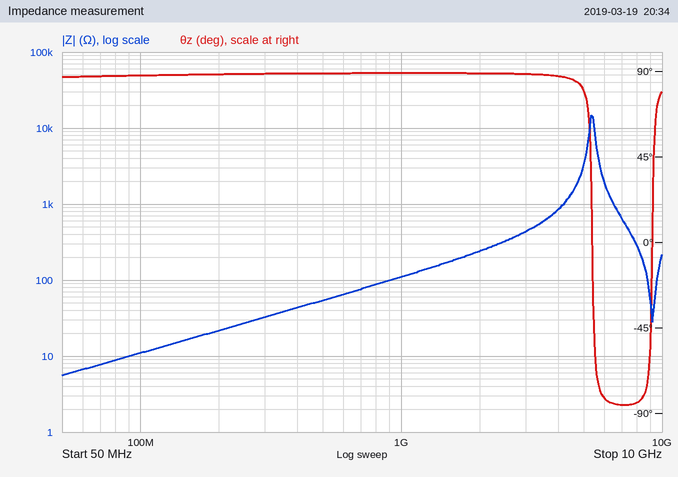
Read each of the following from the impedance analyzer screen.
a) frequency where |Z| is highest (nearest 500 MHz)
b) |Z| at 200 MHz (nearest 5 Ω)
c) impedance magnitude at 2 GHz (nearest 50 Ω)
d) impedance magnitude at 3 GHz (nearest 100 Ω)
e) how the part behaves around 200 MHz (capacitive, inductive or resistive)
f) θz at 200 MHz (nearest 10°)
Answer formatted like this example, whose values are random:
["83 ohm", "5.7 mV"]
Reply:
["5.5 GHz", "20 Ω", "250 Ω", "400 Ω", "inductive", "90°"]
